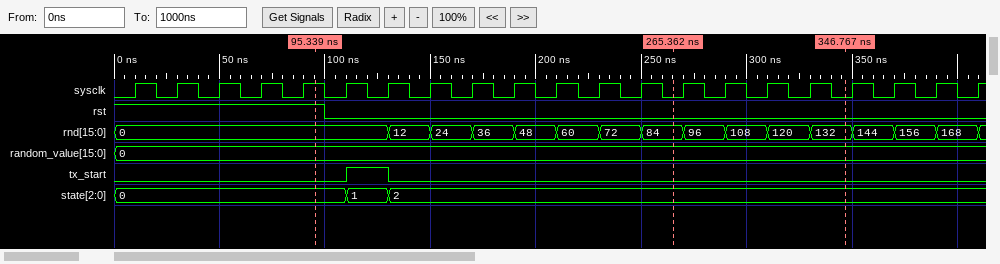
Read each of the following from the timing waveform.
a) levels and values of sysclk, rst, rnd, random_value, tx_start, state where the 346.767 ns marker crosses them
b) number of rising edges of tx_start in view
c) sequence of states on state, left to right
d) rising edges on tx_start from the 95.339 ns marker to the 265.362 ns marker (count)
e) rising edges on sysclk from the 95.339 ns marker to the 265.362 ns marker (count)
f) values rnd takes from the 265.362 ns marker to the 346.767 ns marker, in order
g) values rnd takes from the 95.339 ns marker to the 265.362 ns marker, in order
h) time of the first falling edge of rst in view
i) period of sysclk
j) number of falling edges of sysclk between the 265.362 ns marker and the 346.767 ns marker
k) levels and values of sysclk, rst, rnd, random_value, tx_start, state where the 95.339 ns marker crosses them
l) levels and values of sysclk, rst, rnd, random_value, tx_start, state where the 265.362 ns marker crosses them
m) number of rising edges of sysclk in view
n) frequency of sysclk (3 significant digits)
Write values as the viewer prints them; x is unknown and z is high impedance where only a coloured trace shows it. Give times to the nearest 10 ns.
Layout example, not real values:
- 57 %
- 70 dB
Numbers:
- sysclk=0, rst=0, rnd=132, random_value=0, tx_start=0, state=2
- 1
- 0, 1, 2
- 1
- 8
- 84, 96, 108, 120, 132
- 0, 12, 24, 36, 48, 60, 72, 84
- 100 ns
- 20 ns
- 4
- sysclk=1, rst=1, rnd=0, random_value=0, tx_start=0, state=0
- sysclk=0, rst=0, rnd=84, random_value=0, tx_start=0, state=2
- 21
- 50.0 MHz
